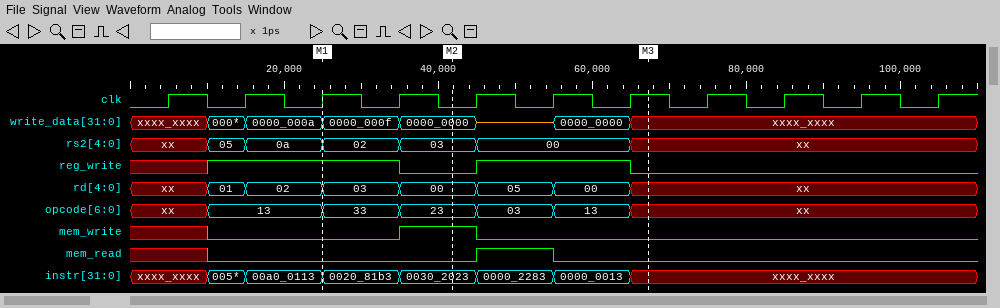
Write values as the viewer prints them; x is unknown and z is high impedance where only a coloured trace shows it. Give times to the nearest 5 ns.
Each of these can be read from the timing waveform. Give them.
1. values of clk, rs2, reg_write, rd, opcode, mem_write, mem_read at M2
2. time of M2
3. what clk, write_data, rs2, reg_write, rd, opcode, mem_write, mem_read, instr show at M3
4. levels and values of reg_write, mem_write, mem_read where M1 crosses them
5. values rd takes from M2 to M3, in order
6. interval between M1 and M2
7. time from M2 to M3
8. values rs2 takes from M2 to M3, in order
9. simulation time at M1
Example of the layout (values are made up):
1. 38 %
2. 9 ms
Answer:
1. clk=0, rs2=03, reg_write=0, rd=00, opcode=23, mem_write=1, mem_read=0
2. 40 ns
3. clk=1, write_data=xxxx_xxxx, rs2=xx, reg_write=0, rd=xx, opcode=xx, mem_write=0, mem_read=0, instr=xxxx_xxxx
4. reg_write=1, mem_write=0, mem_read=0
5. 00, 05, 00, xx
6. 15 ns
7. 25 ns
8. 03, 00, xx
9. 25 ns
